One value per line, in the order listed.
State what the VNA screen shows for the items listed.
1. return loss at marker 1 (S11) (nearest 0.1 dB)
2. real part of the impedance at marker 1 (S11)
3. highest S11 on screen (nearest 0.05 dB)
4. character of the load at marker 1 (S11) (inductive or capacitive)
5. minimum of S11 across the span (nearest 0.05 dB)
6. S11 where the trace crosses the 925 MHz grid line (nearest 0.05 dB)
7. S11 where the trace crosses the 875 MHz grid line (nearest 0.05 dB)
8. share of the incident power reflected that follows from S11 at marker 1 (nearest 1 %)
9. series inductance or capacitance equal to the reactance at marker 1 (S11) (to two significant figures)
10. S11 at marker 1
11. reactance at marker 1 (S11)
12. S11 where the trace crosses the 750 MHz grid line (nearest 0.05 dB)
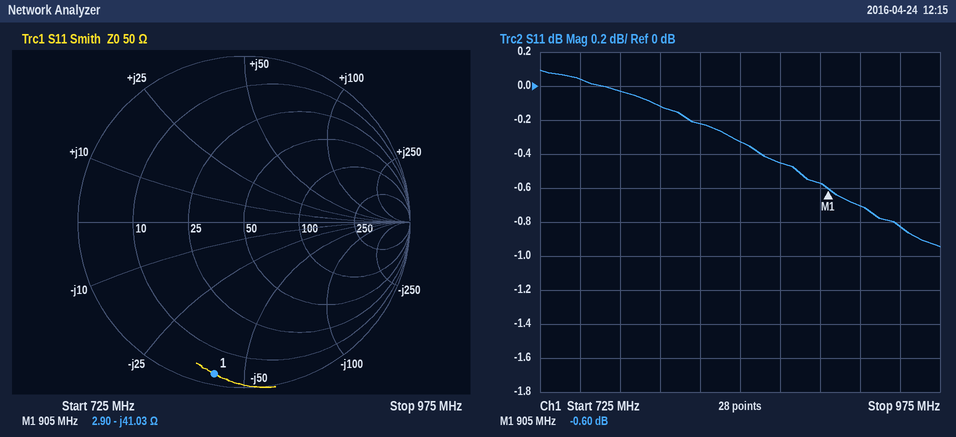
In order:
0.6 dB
2.90 Ω
0.10 dB
capacitive
-0.95 dB
-0.70 dB
-0.45 dB
87 %
4.3 pF
-0.60 dB
-41.03 Ω
0.05 dB
